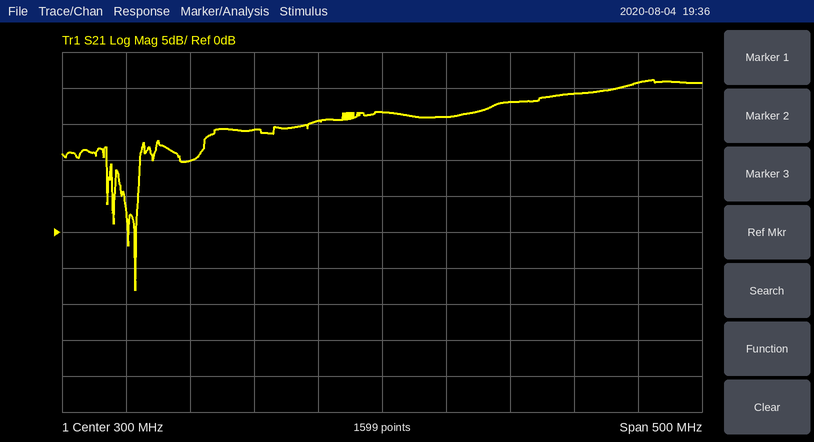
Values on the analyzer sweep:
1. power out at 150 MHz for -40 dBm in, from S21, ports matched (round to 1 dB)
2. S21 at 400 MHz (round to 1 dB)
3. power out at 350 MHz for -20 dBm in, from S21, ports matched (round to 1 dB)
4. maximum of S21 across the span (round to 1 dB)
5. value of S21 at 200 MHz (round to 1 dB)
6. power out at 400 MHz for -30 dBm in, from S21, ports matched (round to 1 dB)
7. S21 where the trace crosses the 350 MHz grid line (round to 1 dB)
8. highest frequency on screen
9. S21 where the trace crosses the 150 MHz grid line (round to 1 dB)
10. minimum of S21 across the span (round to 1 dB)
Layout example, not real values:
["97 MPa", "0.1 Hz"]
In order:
["-30 dBm", "18 dB", "-4 dBm", "21 dB", "14 dB", "-12 dBm", "16 dB", "550 MHz", "10 dB", "-8 dB"]
